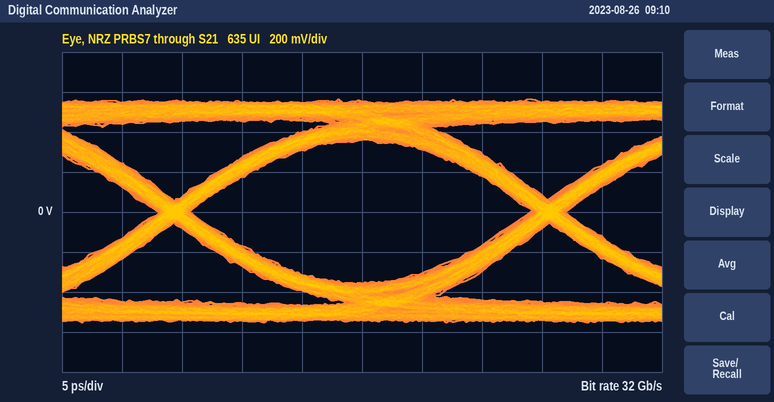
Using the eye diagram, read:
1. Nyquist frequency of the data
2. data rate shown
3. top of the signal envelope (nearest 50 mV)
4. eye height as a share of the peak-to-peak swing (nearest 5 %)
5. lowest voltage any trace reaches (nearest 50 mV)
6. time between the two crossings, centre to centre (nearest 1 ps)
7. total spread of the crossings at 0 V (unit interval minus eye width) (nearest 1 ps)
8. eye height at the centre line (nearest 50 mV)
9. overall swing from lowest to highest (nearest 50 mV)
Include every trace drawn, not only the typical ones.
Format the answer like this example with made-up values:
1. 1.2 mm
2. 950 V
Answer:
1. 16 GHz
2. 32 Gb/s
3. 550 mV
4. 65 %
5. -550 mV
6. 31 ps
7. 3 ps
8. 700 mV
9. 1.10 V
